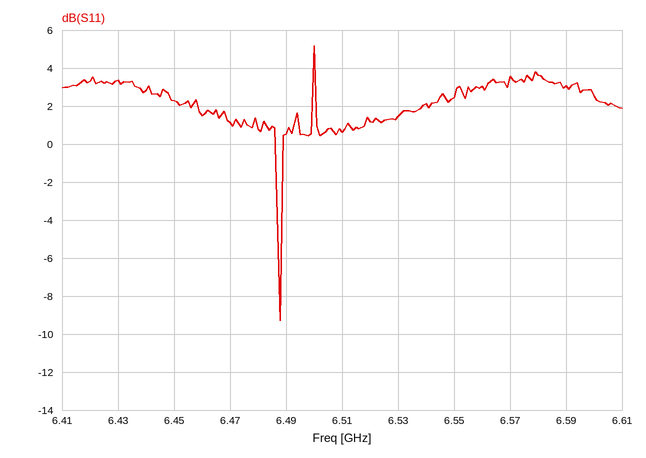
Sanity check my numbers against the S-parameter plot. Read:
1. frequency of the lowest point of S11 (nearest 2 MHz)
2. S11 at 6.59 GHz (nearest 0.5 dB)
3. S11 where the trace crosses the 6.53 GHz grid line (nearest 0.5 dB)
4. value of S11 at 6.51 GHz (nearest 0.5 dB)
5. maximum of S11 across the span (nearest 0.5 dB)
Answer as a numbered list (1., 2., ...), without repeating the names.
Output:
1. 6.488 GHz
2. 3.0 dB
3. 1.5 dB
4. 0.5 dB
5. 5.0 dB
